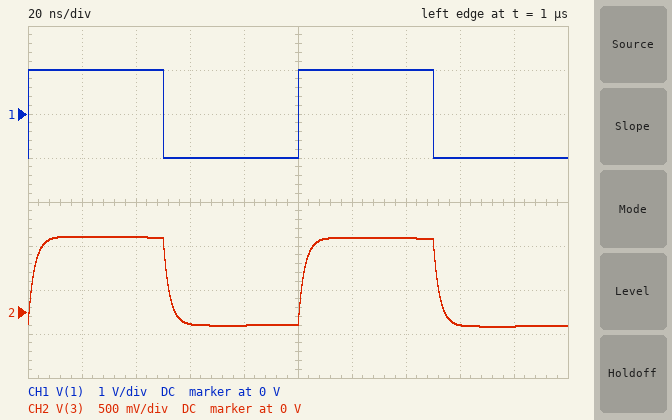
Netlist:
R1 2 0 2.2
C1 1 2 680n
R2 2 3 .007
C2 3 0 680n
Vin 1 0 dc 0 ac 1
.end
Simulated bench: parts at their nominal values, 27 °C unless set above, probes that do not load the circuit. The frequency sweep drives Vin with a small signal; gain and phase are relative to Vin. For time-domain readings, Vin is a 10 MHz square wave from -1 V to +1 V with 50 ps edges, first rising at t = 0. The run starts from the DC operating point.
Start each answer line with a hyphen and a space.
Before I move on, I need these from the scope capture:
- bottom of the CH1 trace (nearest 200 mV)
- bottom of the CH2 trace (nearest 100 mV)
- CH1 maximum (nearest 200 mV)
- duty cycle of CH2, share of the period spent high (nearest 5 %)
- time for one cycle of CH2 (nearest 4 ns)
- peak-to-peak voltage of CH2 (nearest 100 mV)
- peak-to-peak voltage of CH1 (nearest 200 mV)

- -1.0 V
- -200 mV
- 1.0 V
- 50 %
- 100 ns
- 1.0 V
- 2.0 V
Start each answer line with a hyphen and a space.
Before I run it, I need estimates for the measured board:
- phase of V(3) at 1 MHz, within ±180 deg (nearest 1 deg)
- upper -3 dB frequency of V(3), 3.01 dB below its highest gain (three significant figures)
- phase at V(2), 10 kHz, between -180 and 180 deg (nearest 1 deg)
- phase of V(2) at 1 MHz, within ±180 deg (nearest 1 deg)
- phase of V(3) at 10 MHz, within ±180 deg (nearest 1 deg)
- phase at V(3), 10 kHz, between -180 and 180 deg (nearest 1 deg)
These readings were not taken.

- 2 deg
- 67.0 MHz
- 79 deg
- 4 deg
- -8 deg
- 79 deg
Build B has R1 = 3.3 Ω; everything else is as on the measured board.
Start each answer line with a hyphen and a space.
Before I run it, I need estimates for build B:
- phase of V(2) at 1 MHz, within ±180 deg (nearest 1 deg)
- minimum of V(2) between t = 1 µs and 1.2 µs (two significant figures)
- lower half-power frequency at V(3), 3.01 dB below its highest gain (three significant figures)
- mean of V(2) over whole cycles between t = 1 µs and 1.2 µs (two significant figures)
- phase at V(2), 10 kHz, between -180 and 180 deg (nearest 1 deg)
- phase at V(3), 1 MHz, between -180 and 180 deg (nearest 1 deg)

- 3 deg
- -1.1 V
- 35.4 kHz
- 390 mV
- 74 deg
- 1 deg
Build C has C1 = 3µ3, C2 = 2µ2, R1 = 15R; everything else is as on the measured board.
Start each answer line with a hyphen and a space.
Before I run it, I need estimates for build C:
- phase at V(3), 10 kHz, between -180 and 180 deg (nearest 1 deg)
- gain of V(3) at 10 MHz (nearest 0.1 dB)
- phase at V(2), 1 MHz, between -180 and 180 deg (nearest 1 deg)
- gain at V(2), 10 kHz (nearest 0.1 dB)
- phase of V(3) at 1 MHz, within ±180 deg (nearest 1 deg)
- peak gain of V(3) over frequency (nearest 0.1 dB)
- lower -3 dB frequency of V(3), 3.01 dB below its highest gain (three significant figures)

- 11 deg
- -5.7 dB
- 2 deg
- -4.6 dB
- -3 deg
- -4.4 dB
- 1.93 kHz
